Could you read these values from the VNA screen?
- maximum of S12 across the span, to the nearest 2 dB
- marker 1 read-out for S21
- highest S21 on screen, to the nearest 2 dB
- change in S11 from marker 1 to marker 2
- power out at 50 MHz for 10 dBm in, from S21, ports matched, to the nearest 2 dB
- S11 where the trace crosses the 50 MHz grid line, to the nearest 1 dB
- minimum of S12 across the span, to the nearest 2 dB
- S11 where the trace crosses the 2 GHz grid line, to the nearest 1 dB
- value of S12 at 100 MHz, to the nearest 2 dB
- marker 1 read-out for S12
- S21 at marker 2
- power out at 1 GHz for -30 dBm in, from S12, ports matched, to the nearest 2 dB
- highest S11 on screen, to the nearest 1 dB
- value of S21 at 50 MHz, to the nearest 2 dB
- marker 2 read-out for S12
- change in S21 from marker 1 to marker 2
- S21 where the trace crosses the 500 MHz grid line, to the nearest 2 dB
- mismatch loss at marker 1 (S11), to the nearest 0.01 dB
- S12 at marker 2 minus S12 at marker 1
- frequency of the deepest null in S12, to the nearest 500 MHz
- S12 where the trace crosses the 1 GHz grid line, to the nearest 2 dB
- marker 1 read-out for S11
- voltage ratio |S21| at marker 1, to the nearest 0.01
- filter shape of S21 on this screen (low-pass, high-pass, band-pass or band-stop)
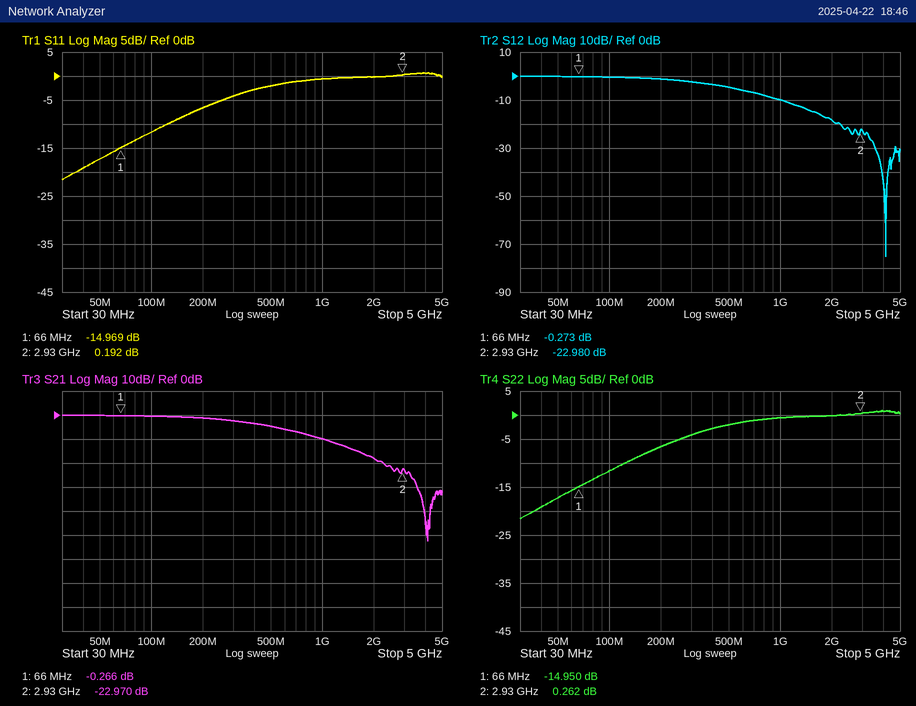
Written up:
0 dB
-0.266 dB
0 dB
15.161 dB
10 dBm
-17 dB
-76 dB
0 dB
0 dB
-0.273 dB
-22.970 dB
-40 dBm
1 dB
0 dB
-22.980 dB
-22.704 dB
-4 dB
0.14 dB
-22.707 dB
4.0 GHz
-10 dB
-14.969 dB
0.97
low-pass
